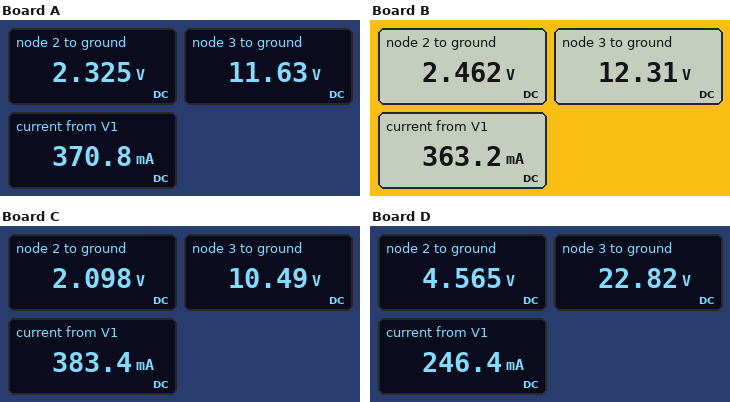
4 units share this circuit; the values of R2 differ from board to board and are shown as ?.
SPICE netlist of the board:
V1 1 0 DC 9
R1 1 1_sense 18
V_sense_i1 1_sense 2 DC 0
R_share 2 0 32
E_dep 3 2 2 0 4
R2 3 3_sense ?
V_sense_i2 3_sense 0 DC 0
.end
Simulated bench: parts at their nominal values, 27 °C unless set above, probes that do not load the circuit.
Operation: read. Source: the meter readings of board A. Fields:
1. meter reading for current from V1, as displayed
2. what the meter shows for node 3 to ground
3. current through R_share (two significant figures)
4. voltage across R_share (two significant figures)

370.8 mA
11.63 V
73 mA
2.3 V
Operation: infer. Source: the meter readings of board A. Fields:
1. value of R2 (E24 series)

39 Ω
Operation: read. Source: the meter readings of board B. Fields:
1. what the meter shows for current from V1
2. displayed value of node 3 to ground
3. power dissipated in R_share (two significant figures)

363.2 mA
12.31 V
190 mW
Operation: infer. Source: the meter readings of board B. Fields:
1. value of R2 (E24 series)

43 Ω
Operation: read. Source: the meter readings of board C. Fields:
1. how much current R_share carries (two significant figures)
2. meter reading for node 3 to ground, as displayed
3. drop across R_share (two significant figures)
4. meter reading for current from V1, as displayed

66 mA
10.49 V
2.1 V
383.4 mA
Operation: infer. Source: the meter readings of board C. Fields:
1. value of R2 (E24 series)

33 Ω
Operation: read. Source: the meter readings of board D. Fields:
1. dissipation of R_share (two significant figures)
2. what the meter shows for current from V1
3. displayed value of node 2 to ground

650 mW
246.4 mA
4.565 V
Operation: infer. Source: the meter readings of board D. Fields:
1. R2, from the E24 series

220 Ω
